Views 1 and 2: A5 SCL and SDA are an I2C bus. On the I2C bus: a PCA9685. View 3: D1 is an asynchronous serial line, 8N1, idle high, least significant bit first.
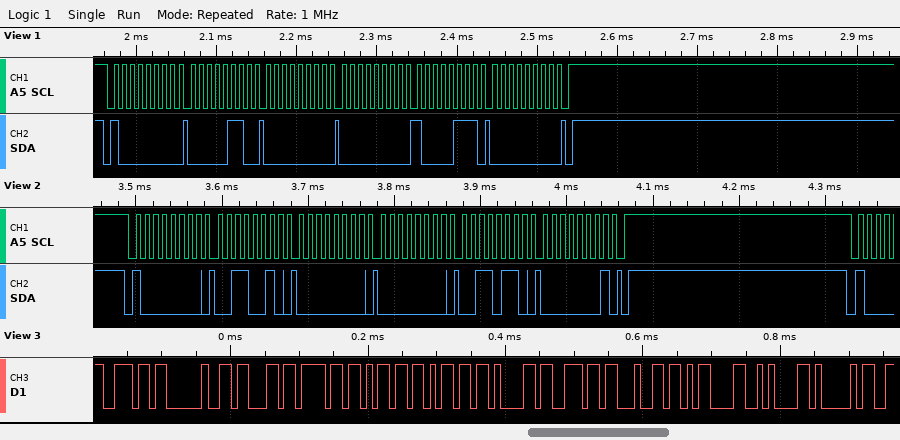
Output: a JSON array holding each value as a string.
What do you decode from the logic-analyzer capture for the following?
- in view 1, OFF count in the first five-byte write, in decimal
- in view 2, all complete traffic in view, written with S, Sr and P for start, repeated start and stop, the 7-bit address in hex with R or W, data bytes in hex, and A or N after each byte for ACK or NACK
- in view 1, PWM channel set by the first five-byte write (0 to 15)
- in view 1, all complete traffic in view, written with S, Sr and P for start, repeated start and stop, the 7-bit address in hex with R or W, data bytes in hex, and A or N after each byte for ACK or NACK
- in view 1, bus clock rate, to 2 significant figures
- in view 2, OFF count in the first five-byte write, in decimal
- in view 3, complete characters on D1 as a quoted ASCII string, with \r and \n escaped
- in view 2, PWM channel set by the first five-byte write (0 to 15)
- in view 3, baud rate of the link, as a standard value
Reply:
["135", "S 40W A 32 A 00 A 00 A 36 A 01 A P", "0", "S 40W A 06 A 00 A 00 A 87 A 00 A P", "100 kHz", "310", "\"n command\\r\\nA\"", "11", "115200 baud"]
